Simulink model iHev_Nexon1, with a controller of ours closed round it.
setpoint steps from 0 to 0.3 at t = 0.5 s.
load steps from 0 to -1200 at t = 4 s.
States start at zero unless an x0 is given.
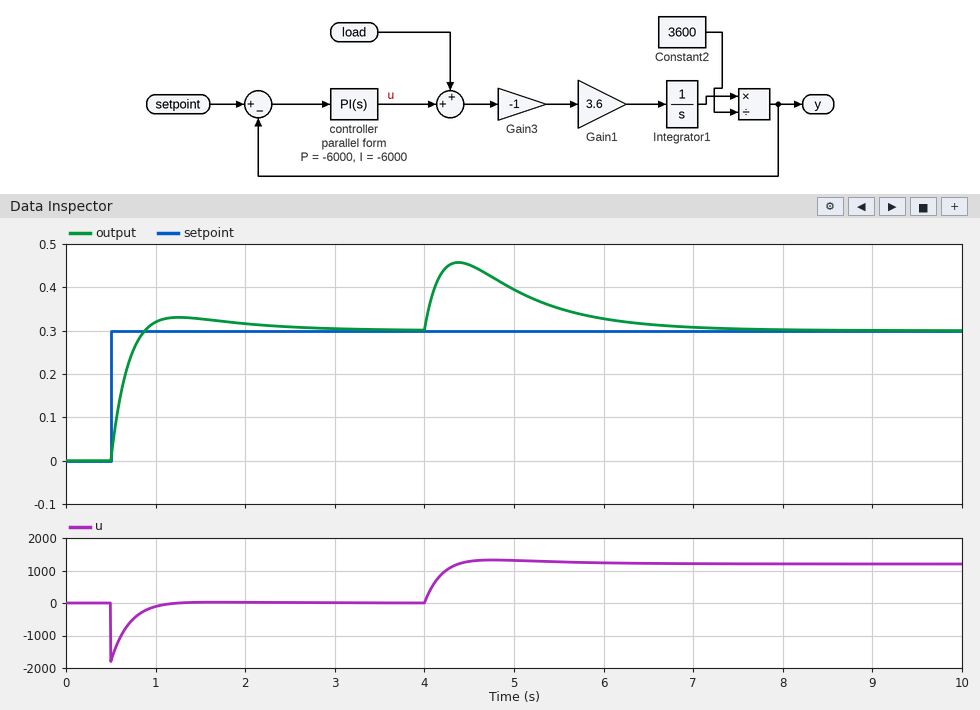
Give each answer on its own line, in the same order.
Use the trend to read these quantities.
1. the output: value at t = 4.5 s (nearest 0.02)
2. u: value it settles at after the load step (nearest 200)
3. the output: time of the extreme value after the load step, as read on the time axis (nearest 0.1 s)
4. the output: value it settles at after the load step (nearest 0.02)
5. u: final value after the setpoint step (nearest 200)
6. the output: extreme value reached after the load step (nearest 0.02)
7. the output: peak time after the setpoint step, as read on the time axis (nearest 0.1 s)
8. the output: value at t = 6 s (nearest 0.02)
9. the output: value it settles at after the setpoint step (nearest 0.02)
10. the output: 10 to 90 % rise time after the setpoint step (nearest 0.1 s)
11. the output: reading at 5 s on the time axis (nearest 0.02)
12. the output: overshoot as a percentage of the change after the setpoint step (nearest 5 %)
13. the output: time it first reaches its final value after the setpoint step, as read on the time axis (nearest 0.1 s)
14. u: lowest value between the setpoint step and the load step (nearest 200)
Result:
0.46
1200
4.4 s
0.30
0
0.46
1.3 s
0.32
0.30
0.3 s
0.40
10 %
0.9 s
-1800
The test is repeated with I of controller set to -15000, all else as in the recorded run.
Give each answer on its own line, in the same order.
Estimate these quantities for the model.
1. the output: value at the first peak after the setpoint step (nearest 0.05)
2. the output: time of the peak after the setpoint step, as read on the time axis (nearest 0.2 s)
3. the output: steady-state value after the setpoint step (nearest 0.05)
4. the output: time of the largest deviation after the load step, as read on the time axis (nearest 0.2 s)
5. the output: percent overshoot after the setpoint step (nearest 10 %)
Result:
0.35
1.0 s
0.30
4.2 s
20 %
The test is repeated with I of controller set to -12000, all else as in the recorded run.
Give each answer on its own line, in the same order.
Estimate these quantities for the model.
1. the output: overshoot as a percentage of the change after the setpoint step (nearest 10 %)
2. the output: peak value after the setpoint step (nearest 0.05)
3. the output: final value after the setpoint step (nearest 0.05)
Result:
20 %
0.35
0.30
